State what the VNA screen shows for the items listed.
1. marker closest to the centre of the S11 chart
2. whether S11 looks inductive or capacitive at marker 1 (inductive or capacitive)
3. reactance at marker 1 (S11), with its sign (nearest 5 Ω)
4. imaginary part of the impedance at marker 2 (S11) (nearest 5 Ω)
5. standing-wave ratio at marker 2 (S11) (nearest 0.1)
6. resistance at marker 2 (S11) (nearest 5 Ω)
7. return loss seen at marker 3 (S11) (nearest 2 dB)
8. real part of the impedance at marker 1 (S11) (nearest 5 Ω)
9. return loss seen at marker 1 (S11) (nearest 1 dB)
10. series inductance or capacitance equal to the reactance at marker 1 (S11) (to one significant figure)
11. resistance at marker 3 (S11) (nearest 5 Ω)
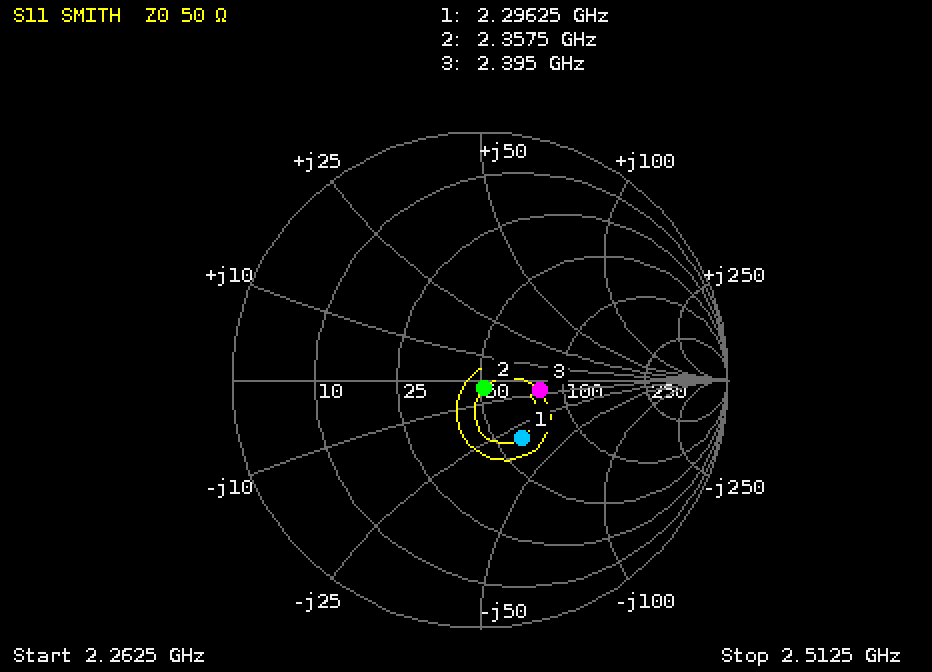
marker 2
capacitive
-30 Ω
-5 Ω
1.1
50 Ω
12 dB
60 Ω
11 dB
2 pF
80 Ω
